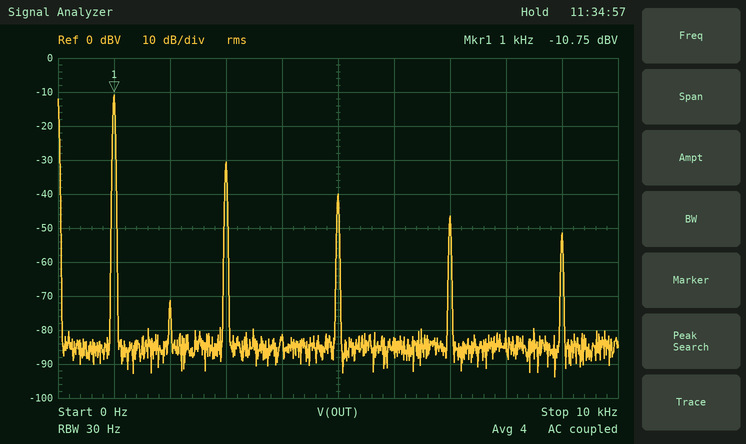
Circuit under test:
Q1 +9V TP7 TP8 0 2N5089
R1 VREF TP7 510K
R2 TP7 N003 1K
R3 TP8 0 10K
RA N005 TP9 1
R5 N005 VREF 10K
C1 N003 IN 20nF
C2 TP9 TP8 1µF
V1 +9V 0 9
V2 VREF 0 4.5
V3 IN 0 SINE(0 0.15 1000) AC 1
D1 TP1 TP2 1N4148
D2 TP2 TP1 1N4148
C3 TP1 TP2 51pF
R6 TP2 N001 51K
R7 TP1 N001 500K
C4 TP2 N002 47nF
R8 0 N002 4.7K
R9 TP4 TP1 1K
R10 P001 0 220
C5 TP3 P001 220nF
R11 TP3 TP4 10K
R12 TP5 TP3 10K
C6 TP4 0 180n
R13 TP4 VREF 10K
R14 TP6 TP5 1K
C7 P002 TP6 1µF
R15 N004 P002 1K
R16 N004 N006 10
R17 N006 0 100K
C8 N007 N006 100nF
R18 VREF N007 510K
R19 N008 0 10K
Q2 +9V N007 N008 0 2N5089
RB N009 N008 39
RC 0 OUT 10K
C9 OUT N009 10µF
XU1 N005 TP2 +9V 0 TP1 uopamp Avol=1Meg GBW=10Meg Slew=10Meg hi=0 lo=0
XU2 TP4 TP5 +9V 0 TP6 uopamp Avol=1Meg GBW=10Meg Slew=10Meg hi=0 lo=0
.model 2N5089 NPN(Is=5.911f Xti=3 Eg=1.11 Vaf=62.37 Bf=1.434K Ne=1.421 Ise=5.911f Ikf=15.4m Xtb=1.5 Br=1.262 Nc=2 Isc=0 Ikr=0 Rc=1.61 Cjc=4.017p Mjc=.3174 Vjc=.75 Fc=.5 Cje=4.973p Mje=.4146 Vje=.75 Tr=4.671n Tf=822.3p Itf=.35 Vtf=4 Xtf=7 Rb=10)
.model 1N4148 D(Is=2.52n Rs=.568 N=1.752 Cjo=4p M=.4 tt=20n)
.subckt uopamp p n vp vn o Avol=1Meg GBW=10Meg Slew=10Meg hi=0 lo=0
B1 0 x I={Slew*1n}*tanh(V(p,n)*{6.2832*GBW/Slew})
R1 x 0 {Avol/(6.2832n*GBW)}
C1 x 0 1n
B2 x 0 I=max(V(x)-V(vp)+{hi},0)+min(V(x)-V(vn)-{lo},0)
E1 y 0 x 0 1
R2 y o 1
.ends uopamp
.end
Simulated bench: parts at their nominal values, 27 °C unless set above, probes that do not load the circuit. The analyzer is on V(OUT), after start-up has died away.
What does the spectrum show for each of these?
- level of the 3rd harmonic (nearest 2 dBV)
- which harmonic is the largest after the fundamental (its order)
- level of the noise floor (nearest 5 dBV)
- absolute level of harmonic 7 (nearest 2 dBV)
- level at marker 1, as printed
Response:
-30 dBV
3
-85 dBV
-46 dBV
-10.75 dBV
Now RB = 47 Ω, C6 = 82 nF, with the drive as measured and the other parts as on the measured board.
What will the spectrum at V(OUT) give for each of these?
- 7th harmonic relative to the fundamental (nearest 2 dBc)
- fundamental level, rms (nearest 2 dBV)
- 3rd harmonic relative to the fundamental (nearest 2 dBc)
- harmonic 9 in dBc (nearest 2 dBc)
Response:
-32 dBc
-8 dBV
-16 dBc
-36 dBc
